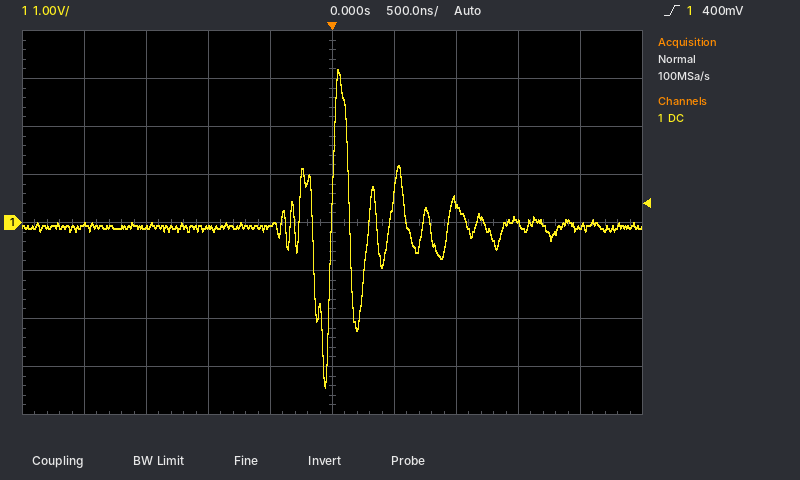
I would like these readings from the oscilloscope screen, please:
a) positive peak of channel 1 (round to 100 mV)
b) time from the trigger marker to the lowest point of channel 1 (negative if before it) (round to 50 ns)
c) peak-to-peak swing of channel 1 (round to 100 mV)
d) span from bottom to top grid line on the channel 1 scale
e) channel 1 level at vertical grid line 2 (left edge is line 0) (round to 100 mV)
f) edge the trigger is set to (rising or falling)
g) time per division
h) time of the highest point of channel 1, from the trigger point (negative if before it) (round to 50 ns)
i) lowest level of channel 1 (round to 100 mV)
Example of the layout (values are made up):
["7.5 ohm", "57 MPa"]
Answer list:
["3.2 V", "-50 ns", "6.6 V", "8 V", "-100 mV", "rising", "500 ns", "+50 ns", "-3.4 V"]
